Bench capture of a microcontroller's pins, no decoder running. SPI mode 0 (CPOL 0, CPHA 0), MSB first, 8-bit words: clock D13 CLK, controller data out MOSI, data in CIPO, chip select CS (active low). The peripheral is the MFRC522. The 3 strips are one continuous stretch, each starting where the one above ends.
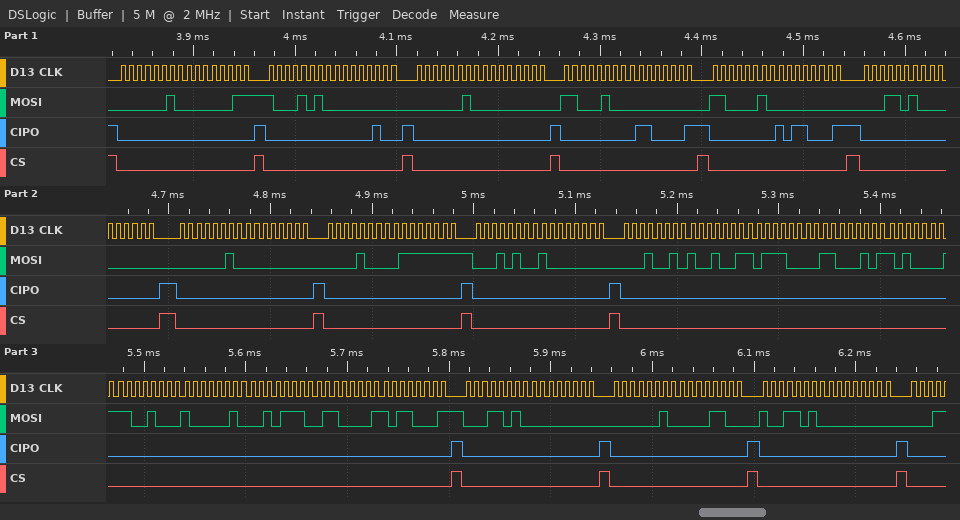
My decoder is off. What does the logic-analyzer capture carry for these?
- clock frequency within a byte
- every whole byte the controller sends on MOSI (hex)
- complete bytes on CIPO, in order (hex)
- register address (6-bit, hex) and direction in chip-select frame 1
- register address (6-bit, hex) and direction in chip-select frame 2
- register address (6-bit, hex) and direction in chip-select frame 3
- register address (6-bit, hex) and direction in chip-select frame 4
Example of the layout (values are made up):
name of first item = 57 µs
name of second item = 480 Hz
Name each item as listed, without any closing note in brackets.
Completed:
clock frequency within a byte = 125 kHz
every whole byte the controller sends on MOSI = 02 03 8A 00 02 00 C4 00 C2 00 1A 00 02 00 08 7F 14 80 12 93 70 C5 A1 C8 82 2E 61 B1 1A 00 02 0C 9A 00
complete bytes on CIPO, in order = 00 00 00 04 00 00 00 61 00 B1 00 00 00 00 00 00 00 00 00 00 00 00 00 00 00 00 00 00 00 00 00 00 00 00
register address (6-bit, hex) and direction in chip-select frame 1 = 0x01 write
register address (6-bit, hex) and direction in chip-select frame 2 = 0x05 read
register address (6-bit, hex) and direction in chip-select frame 3 = 0x01 write
register address (6-bit, hex) and direction in chip-select frame 4 = 0x22 read
